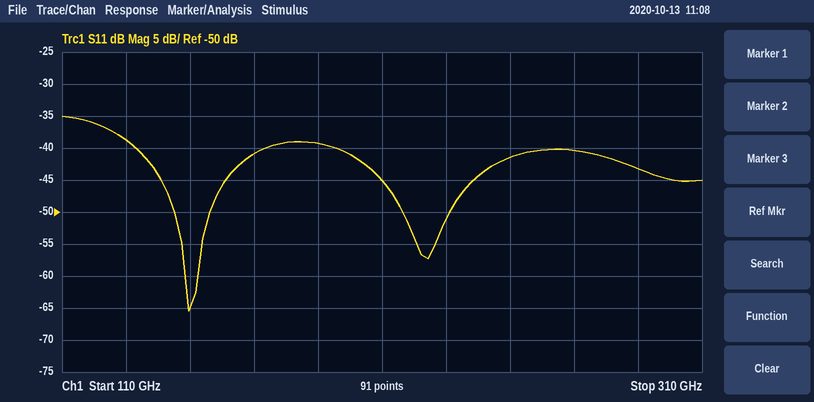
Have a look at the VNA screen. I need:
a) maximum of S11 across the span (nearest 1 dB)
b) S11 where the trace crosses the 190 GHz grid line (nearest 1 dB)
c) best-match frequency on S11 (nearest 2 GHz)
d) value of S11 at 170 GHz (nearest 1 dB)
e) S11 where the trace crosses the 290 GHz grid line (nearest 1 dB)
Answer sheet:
-35 dB
-39 dB
150 GHz
-41 dB
-43 dB
